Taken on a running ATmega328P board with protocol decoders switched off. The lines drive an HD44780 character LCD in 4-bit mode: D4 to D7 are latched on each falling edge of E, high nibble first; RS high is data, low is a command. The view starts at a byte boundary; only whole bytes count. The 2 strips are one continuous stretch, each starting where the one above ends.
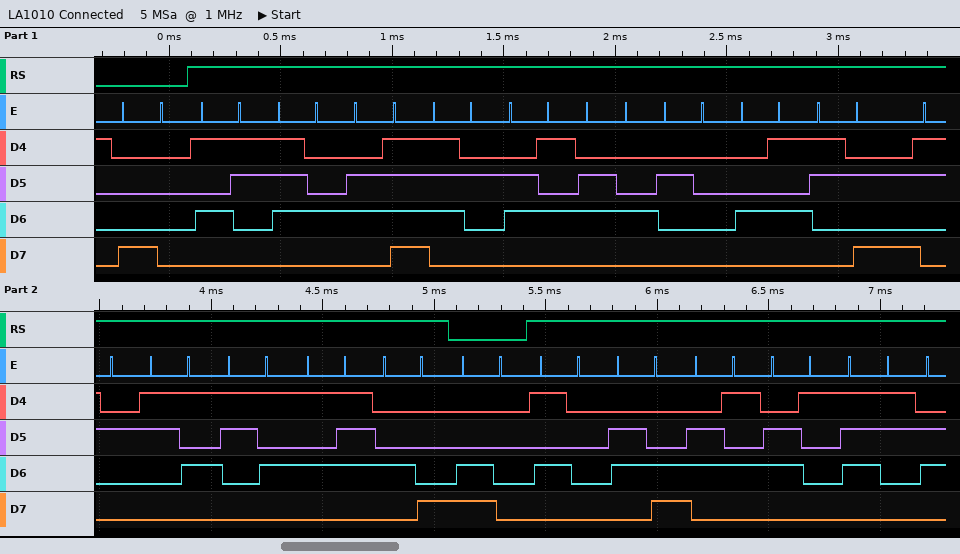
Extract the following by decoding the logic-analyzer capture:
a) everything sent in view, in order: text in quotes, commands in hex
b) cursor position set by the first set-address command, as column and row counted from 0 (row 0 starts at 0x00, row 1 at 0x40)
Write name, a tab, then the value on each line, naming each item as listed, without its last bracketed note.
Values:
everything sent in view, in order: text in quotes, commands in hex	0x80 "Stored E:255WH" 0xC0 "Pleas"
cursor position set by the first set-address command, as column and row counted from 0	column 0, row 0
